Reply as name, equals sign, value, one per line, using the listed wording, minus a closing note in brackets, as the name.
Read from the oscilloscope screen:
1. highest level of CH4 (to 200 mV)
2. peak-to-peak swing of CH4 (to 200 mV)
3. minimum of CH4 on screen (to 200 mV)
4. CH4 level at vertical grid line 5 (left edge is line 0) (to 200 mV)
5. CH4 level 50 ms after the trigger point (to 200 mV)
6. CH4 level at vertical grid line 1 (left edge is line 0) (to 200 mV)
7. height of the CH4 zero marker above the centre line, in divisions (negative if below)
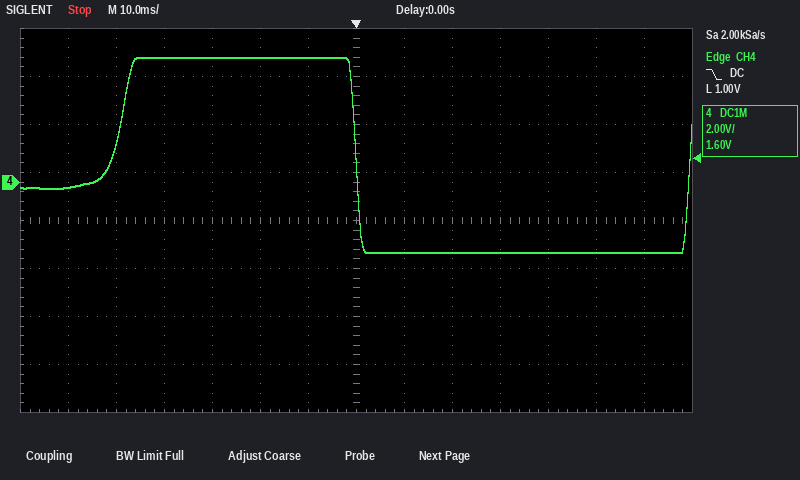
highest level of CH4 = 5.2 V
peak-to-peak swing of CH4 = 8.2 V
minimum of CH4 on screen = -3.0 V
CH4 level at vertical grid line 5 (left edge is line 0) = 5.2 V
CH4 level 50 ms after the trigger point = -3.0 V
CH4 level at vertical grid line 1 (left edge is line 0) = -200 mV
height of the CH4 zero marker above the centre line, in divisions = +0.8 div
